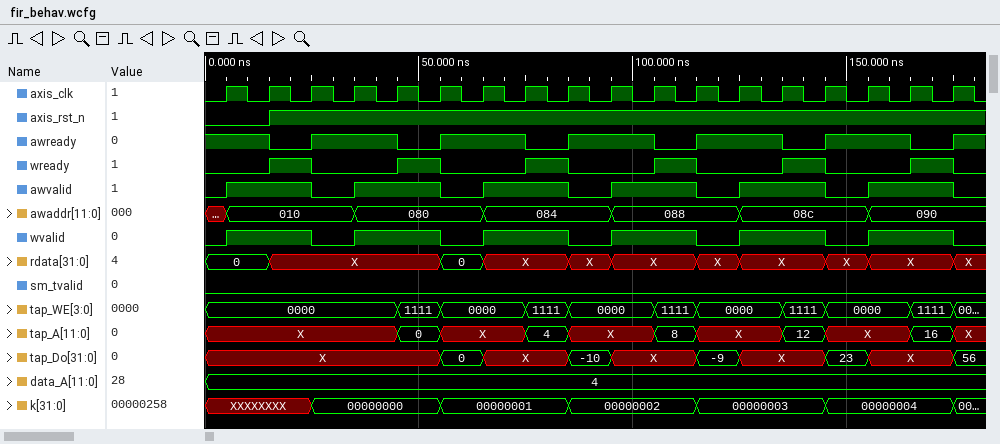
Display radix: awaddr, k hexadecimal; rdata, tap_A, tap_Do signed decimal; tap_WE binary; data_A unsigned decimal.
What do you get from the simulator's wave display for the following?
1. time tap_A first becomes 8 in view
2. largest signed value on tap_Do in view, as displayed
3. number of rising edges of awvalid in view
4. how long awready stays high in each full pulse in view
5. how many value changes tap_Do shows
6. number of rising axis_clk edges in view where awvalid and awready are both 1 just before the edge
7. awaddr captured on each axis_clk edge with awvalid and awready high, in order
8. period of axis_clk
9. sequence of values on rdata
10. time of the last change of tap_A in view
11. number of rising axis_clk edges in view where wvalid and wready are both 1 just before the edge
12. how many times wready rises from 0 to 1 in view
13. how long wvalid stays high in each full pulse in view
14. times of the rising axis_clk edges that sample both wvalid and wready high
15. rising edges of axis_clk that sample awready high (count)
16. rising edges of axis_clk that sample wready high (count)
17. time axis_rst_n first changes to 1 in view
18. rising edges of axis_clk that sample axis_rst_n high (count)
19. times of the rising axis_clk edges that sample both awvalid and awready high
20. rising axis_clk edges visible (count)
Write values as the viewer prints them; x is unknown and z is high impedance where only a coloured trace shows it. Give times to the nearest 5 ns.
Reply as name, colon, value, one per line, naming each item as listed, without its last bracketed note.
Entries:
time tap_A first becomes 8 in view: 105 ns
largest signed value on tap_Do in view, as displayed: 56
number of rising edges of awvalid in view: 6
how long awready stays high in each full pulse in view: 20 ns, 20 ns, 20 ns, 20 ns, 20 ns
how many value changes tap_Do shows: 9
number of rising axis_clk edges in view where awvalid and awready are both 1 just before the edge: 6
awaddr captured on each axis_clk edge with awvalid and awready high, in order: 010, 080, 084, 088, 08c, 090
period of axis_clk: 10 ns
sequence of values on rdata: 0, X, 0, X, X, X, X, X, X, X, X
time of the last change of tap_A in view: 175 ns
number of rising axis_clk edges in view where wvalid and wready are both 1 just before the edge: 6
how many times wready rises from 0 to 1 in view: 6
how long wvalid stays high in each full pulse in view: 20 ns, 20 ns, 20 ns, 20 ns, 20 ns, 20 ns
times of the rising axis_clk edges that sample both wvalid and wready high: 25 ns, 55 ns, 85 ns, 115 ns, 145 ns, 175 ns
rising edges of axis_clk that sample awready high: 12
rising edges of axis_clk that sample wready high: 6
time axis_rst_n first changes to 1 in view: 15 ns
rising edges of axis_clk that sample axis_rst_n high: 16
times of the rising axis_clk edges that sample both awvalid and awready high: 15 ns, 45 ns, 75 ns, 105 ns, 135 ns, 165 ns
rising axis_clk edges visible: 18
